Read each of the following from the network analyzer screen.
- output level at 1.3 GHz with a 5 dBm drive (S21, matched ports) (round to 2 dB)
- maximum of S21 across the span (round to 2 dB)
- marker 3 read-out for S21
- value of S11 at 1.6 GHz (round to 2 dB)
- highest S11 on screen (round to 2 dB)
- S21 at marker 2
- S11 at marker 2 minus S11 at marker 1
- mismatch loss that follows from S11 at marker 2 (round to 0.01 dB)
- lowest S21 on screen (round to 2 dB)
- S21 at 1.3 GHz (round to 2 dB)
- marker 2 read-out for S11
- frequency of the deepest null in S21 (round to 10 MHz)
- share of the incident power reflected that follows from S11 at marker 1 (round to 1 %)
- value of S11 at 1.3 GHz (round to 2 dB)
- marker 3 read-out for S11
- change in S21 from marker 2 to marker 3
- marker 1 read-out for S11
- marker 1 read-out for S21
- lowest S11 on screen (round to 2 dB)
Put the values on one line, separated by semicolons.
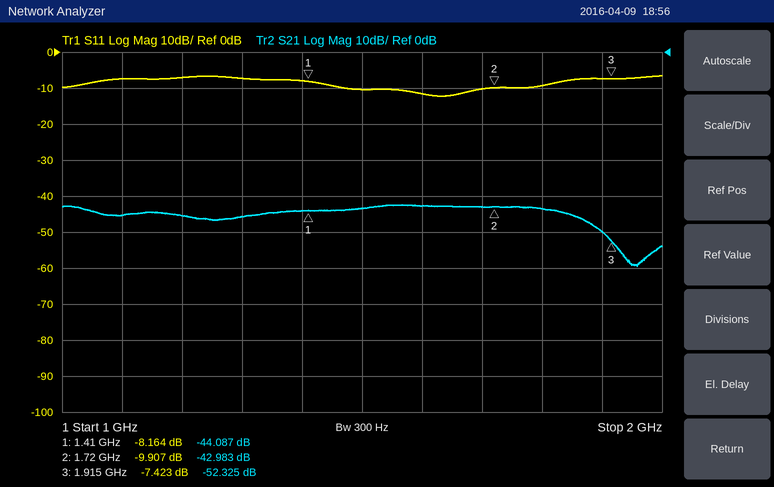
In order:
-40 dBm; -42 dB; -52.325 dB; -12 dB; -6 dB; -42.983 dB; -1.743 dB; 0.47 dB; -60 dB; -46 dB; -9.907 dB; 1.96 GHz; 15 %; -8 dB; -7.423 dB; -9.342 dB; -8.164 dB; -44.087 dB; -12 dB
